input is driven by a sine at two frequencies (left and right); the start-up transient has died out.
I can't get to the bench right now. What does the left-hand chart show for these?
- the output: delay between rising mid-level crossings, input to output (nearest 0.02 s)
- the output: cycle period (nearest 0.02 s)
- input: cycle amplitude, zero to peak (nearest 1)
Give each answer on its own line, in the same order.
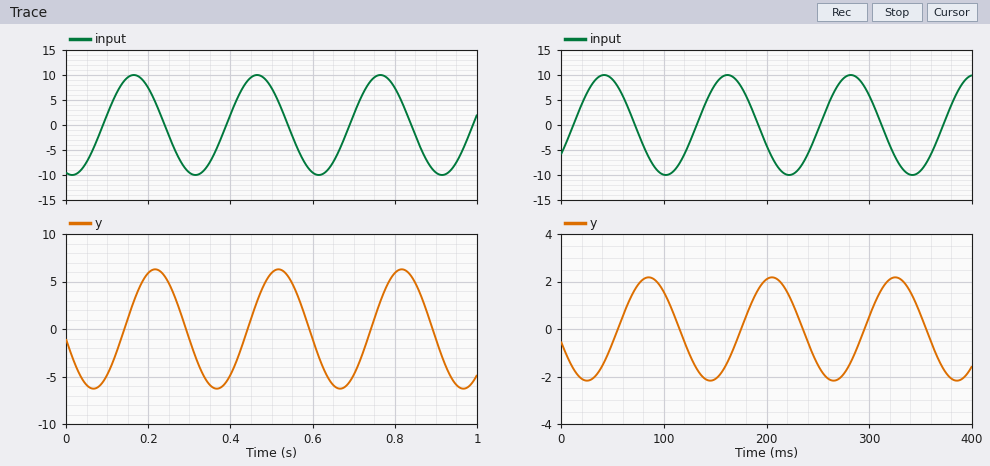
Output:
0.06 s
0.30 s
10
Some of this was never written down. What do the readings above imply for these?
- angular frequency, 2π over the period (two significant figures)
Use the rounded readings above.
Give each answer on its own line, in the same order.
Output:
21 rad/s
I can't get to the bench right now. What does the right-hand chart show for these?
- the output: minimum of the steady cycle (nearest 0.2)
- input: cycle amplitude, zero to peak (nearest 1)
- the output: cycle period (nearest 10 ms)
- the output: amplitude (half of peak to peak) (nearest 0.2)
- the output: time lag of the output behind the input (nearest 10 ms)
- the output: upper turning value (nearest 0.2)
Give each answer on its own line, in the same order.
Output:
-2.2
10
120 ms
2.2
40 ms
2.2
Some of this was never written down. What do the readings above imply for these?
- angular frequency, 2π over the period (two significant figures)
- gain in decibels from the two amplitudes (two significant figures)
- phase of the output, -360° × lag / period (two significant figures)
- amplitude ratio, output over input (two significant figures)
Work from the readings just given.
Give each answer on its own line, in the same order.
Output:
0.052 rad/ms
-13 dB
-120°
0.22
